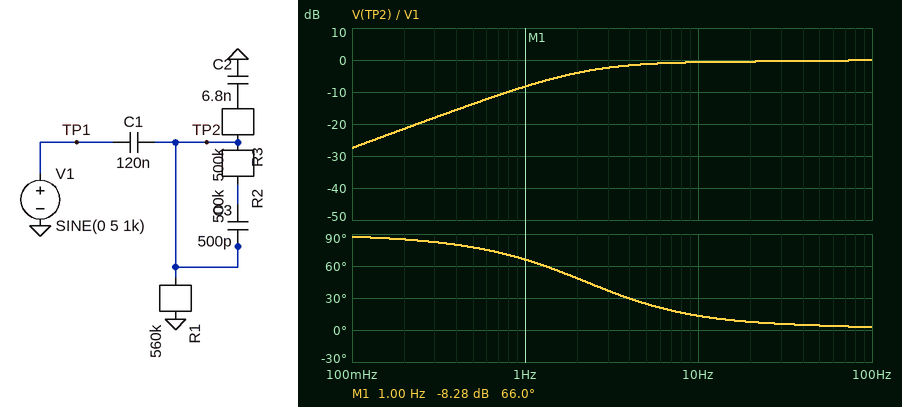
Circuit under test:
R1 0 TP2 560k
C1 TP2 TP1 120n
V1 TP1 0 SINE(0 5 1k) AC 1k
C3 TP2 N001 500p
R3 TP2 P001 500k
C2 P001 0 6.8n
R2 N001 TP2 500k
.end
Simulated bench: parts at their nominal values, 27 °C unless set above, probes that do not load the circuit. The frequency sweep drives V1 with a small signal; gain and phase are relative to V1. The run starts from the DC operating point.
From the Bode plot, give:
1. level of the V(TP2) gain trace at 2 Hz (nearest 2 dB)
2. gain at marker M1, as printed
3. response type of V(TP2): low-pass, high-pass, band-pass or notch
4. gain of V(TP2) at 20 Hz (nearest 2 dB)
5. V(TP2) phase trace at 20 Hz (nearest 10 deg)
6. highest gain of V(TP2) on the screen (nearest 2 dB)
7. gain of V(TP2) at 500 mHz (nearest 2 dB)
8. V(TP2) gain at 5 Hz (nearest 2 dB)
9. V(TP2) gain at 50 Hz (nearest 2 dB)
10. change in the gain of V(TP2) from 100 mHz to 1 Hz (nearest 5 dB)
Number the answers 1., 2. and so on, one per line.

1. -4 dB
2. -8.28 dB
3. high-pass
4. 0 dB
5. 10 deg
6. 0 dB
7. -14 dB
8. -2 dB
9. 0 dB
10. 20 dB
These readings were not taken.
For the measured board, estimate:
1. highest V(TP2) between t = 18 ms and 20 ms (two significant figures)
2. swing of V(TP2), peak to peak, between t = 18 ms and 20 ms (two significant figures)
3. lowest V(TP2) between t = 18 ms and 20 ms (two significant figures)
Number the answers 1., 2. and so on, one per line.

1. 5.0 V
2. 10 V
3. -5.0 V
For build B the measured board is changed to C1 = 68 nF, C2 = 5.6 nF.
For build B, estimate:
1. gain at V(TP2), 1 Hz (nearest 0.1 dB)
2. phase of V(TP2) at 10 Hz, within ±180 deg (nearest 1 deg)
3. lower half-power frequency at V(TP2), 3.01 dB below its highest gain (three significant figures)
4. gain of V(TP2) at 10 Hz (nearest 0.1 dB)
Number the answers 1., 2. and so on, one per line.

1. -12.7 dB
2. 22 deg
3. 4.62 Hz
4. -1.3 dB
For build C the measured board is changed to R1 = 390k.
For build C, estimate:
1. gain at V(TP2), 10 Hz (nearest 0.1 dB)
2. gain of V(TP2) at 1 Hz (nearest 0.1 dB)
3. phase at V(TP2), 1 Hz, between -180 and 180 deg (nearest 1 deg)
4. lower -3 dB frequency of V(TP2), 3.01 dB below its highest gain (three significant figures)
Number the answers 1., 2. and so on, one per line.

1. -0.9 dB
2. -11.0 dB
3. 73 deg
4. 3.63 Hz
